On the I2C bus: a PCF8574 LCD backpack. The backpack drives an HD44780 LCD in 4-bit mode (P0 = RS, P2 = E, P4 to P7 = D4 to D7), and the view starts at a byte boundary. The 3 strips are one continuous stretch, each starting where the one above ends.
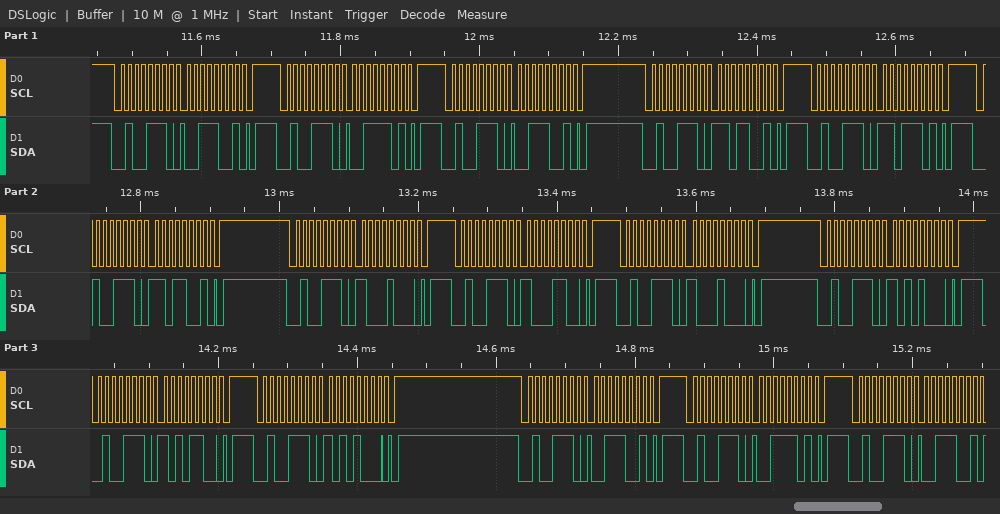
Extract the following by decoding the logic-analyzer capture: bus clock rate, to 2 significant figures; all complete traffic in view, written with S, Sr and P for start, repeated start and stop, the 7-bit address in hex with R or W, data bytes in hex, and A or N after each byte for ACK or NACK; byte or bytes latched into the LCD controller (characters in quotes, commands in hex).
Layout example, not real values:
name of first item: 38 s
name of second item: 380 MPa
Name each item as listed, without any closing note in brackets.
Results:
bus clock rate, to 2 significant figures: 100 kHz
all complete traffic in view, written with S, Sr and P for start, repeated start and stop, the 7-bit address in hex with R or W, data bytes in hex, and A or N after each byte for ACK or NACK: S 27W A 39 A P S 27W A 3D A P S 27W A 39 A P S 27W A D9 A P S 27W A DD A P S 27W A D9 A P S 27W A 88 A P S 27W A 8C A P S 27W A 88 A P S 27W A A8 A P S 27W A AC A P S 27W A A8 A P S 27W A 39 A P S 27W A 3D A P S 27W A 39 A
byte or bytes latched into the LCD controller: '=' 0x8A
